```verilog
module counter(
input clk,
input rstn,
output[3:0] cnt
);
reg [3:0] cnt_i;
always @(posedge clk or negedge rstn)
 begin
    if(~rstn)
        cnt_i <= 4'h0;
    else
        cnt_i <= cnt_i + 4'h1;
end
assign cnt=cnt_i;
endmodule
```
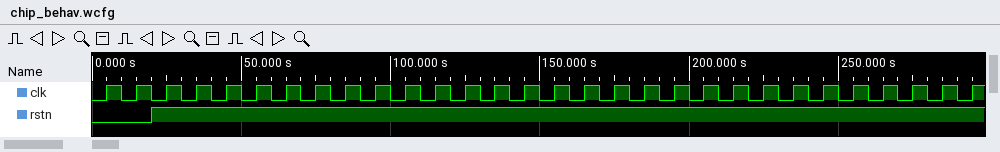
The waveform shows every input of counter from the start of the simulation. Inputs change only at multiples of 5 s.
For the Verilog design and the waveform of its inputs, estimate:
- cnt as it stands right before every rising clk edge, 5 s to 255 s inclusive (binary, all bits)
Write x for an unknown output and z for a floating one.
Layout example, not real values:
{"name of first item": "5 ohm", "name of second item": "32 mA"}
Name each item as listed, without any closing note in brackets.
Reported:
{"cnt as it stands right before every rising clk edge, 5 s to 255 s inclusive": "0000, 0000, 0000, 0001, 0010, 0011, 0100, 0101, 0110, 0111, 1000, 1001, 1010, 1011, 1100, 1101, 1110, 1111, 0000, 0001, 0010, 0011, 0100, 0101, 0110, 0111"}
